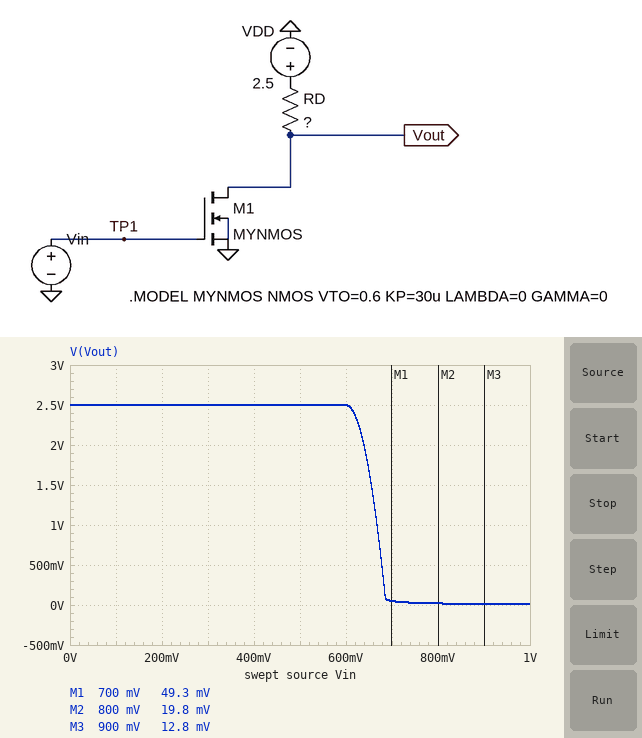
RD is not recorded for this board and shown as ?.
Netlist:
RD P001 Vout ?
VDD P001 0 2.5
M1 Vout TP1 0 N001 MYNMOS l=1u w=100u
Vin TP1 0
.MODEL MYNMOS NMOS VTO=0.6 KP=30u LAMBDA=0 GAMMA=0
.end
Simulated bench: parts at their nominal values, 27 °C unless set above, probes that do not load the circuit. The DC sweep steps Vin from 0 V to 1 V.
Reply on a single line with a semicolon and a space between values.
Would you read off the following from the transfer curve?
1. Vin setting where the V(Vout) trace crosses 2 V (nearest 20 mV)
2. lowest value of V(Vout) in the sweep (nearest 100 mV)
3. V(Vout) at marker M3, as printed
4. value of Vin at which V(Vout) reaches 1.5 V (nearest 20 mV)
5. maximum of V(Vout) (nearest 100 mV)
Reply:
640 mV; 0 V; 12.8 mV; 660 mV; 2.5 V
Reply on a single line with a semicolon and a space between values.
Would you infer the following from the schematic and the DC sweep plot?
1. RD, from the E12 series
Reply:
220 kΩ
